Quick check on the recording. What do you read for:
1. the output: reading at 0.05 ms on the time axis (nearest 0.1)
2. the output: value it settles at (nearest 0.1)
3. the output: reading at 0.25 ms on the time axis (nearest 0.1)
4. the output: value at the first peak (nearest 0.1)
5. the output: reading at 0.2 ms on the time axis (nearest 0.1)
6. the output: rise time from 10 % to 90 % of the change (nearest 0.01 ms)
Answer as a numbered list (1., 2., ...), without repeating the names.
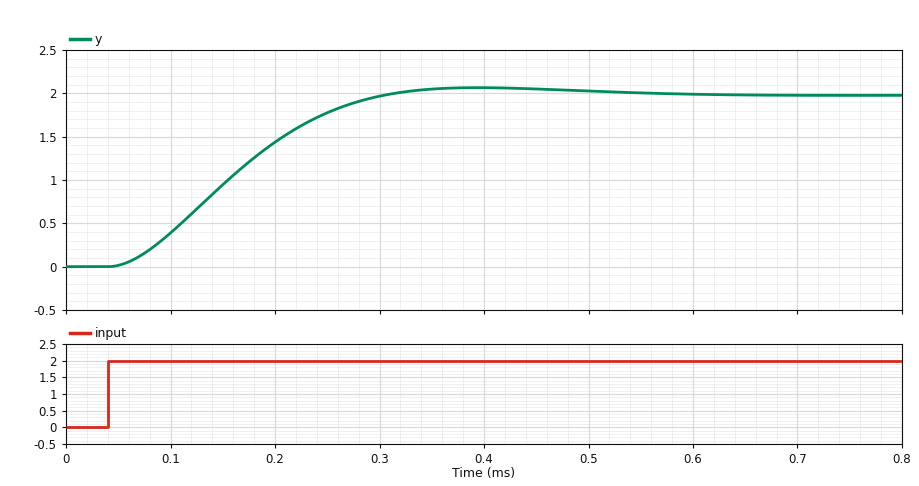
1. 0.0
2. 2.0
3. 1.8
4. 2.1
5. 1.4
6. 0.17 ms
